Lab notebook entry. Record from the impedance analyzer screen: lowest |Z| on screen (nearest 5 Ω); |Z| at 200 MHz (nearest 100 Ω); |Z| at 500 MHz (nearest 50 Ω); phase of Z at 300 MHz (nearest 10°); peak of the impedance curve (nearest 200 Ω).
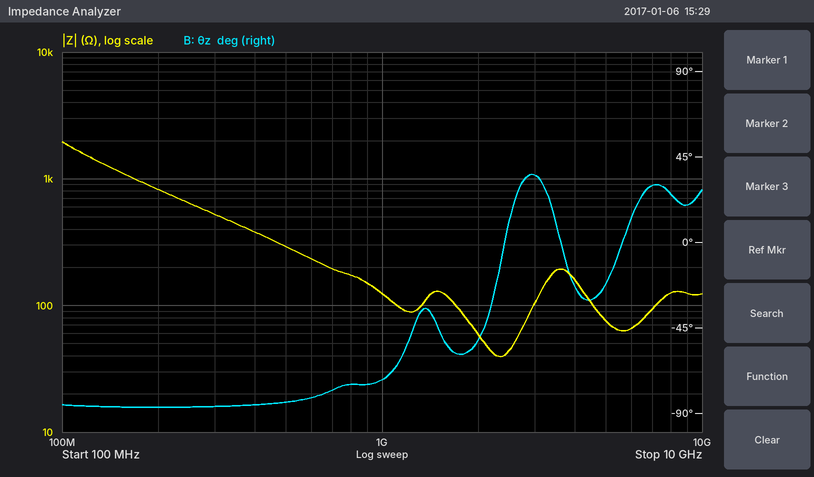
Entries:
40 Ω
800 Ω
300 Ω
-90°
2.0 kΩ
